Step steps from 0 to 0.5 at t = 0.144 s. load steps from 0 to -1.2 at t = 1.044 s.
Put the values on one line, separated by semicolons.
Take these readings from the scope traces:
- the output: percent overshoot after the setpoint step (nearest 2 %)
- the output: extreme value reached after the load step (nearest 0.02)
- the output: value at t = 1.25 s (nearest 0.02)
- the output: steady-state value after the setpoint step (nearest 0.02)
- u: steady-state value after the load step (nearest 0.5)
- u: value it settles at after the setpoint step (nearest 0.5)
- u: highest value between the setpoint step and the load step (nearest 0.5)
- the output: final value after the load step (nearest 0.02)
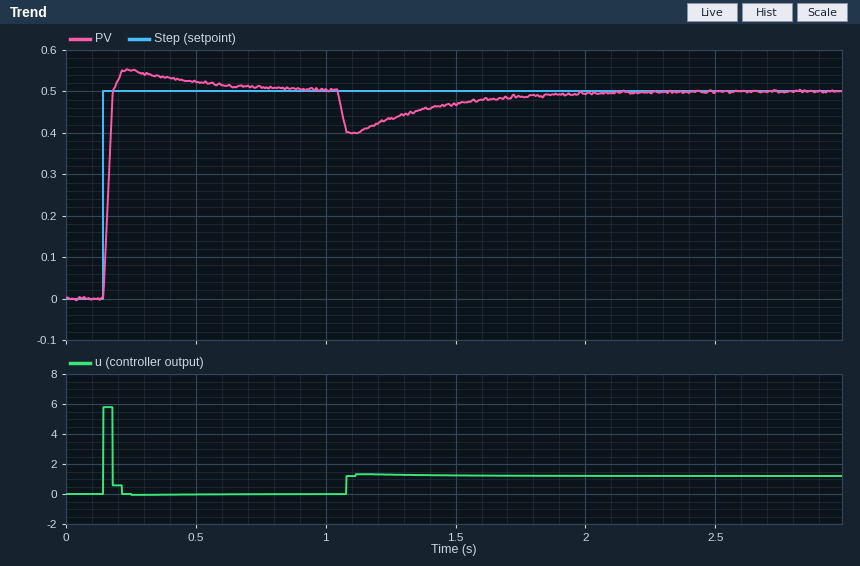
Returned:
10 %; 0.40; 0.44; 0.50; 1.0; 0.0; 6.0; 0.50
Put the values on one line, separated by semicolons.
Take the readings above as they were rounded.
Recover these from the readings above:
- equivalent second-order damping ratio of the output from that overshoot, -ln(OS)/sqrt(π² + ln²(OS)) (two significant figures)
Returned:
0.59
